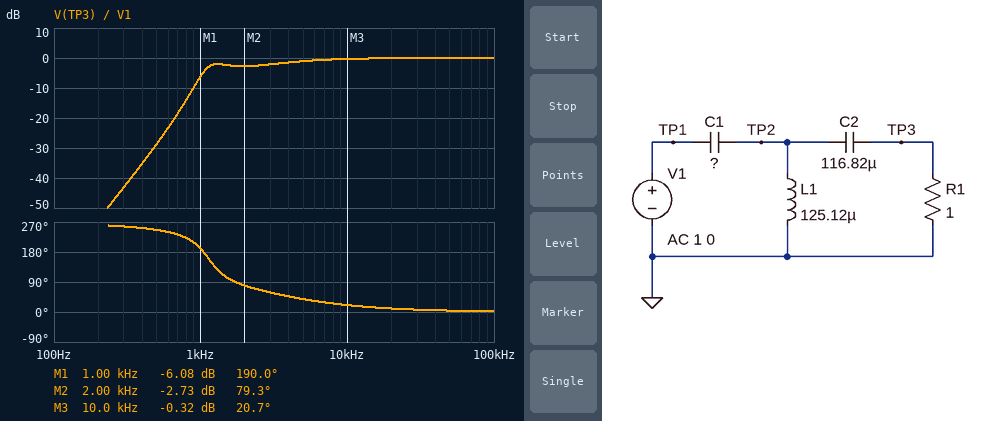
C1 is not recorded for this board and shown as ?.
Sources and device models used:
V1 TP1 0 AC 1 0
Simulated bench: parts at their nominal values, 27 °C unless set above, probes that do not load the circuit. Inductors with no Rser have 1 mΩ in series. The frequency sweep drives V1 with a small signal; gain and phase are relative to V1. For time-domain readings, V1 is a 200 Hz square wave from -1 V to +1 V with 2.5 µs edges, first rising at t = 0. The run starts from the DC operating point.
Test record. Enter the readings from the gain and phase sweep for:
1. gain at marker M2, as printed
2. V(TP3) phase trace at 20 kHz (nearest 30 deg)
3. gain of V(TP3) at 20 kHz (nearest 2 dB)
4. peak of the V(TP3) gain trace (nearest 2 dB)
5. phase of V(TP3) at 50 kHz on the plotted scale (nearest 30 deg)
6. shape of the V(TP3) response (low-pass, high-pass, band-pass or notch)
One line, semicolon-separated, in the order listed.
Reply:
-2.73 dB; 0 deg; 0 dB; 0 dB; 0 deg; high-pass
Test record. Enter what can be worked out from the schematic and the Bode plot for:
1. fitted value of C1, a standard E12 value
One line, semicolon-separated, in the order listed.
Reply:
68 µF
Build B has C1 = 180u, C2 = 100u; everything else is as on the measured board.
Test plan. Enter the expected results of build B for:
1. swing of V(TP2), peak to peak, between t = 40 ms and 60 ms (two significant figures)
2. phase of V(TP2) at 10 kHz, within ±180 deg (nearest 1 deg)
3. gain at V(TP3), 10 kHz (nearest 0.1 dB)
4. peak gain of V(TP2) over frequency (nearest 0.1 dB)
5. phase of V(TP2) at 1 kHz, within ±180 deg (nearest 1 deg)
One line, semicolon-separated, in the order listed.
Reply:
3.7 V; 5 deg; -0.2 dB; 12.5 dB; 43 deg
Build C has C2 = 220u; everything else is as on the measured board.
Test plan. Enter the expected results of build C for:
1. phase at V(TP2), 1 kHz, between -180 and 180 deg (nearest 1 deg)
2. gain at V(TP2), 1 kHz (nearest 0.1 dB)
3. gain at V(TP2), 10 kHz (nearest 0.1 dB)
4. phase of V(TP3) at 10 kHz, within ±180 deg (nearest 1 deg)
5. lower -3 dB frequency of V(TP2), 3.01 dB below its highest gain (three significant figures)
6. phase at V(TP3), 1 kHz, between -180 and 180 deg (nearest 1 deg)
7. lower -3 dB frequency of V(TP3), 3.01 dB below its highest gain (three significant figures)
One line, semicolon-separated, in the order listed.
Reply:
119 deg; -4.9 dB; -0.1 dB; 17 deg; 1.24 kHz; 155 deg; 1.56 kHz
